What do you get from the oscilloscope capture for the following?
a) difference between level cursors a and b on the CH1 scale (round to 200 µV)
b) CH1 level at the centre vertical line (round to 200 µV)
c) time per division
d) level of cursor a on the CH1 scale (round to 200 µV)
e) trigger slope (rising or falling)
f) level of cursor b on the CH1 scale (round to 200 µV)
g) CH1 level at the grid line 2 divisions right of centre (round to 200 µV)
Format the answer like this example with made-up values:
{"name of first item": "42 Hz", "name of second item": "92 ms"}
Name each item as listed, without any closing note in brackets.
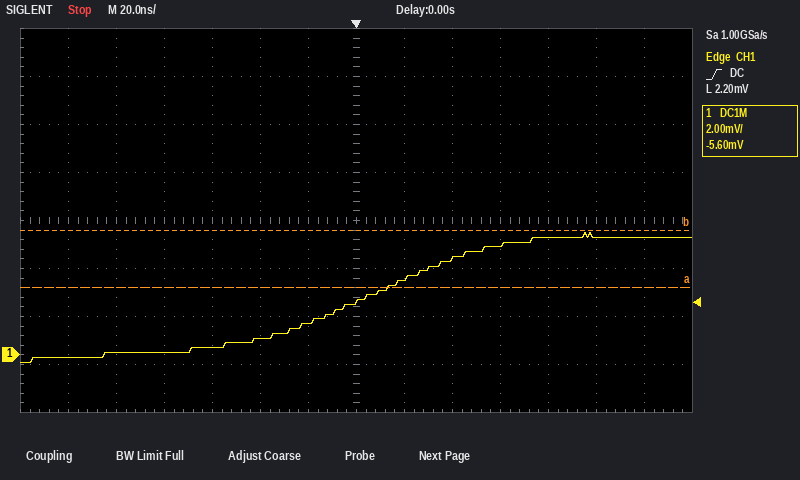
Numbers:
{"difference between level cursors a and b on the CH1 scale": "2.4 mV", "CH1 level at the centre vertical line": "2.2 mV", "time per division": "20 ns", "level of cursor a on the CH1 scale": "2.8 mV", "trigger slope": "rising", "level of cursor b on the CH1 scale": "5.2 mV", "CH1 level at the grid line 2 divisions right of centre": "4.0 mV"}
